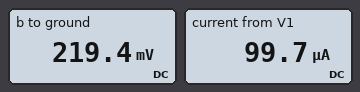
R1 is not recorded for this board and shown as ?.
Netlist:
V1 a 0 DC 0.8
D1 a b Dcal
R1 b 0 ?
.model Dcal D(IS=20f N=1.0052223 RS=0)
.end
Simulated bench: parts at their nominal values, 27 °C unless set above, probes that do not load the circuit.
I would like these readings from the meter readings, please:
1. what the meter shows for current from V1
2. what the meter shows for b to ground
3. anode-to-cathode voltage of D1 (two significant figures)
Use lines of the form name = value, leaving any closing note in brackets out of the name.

what the meter shows for current from V1 = 99.7 µA
what the meter shows for b to ground = 219.4 mV
anode-to-cathode voltage of D1 = 580 mV
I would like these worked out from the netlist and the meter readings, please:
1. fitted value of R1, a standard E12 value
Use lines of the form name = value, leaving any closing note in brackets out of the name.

fitted value of R1, a standard E12 value = 2.2 kΩ
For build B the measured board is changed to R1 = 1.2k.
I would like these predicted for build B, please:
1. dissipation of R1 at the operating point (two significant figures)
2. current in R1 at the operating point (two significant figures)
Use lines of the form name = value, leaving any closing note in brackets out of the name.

dissipation of R1 at the operating point = 35 µW
current in R1 at the operating point = 170 µA
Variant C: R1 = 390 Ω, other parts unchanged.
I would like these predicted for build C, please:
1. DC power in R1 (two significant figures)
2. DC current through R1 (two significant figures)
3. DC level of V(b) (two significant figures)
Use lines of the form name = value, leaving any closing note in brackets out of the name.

DC power in R1 = 83 µW
DC current through R1 = 460 µA
DC level of V(b) = 180 mV
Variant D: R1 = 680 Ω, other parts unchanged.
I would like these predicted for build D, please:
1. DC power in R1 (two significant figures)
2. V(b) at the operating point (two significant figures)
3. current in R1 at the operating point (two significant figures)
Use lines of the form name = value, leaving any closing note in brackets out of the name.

DC power in R1 = 54 µW
V(b) at the operating point = 190 mV
current in R1 at the operating point = 280 µA
